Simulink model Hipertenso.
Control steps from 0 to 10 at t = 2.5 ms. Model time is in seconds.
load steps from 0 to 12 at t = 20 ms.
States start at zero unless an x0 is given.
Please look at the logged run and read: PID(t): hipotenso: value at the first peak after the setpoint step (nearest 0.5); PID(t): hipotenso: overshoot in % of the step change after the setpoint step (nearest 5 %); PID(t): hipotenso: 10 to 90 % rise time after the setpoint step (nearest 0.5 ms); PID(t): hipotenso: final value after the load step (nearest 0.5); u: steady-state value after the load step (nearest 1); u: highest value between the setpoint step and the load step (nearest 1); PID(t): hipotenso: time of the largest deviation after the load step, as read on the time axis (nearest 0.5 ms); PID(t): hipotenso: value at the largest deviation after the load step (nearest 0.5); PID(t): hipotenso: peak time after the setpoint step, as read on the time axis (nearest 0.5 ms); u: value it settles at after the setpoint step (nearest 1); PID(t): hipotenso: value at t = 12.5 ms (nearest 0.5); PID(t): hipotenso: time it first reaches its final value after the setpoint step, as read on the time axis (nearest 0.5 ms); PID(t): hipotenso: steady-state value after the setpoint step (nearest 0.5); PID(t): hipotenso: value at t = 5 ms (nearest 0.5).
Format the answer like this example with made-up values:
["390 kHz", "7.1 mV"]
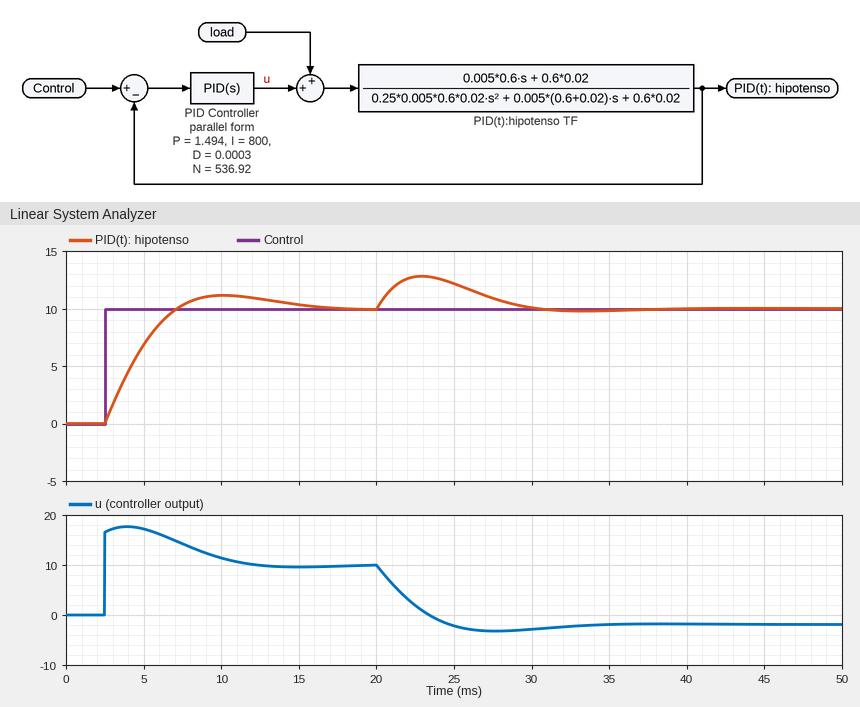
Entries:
["11.0", "10 %", "3.5 ms", "10.0", "-2", "18", "23.0 ms", "13.0", "10.0 ms", "10", "11.0", "7.0 ms", "10.0", "7.0"]
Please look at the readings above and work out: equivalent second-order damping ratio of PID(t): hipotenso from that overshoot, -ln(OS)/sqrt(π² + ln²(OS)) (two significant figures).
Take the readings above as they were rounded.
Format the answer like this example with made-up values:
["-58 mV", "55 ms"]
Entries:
["0.59"]
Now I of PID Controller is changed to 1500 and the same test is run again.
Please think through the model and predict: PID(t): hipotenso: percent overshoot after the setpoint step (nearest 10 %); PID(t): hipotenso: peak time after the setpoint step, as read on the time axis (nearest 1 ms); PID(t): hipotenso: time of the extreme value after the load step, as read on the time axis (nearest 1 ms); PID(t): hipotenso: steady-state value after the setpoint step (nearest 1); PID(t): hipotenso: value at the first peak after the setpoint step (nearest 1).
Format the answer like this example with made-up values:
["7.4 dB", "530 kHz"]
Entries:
["20 %", "8 ms", "22 ms", "10", "12"]
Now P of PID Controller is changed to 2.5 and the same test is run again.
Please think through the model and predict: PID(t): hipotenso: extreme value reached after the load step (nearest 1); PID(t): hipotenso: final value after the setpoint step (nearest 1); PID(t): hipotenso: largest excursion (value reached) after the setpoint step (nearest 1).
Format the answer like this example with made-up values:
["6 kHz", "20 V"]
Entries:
["12", "10", "10"]
